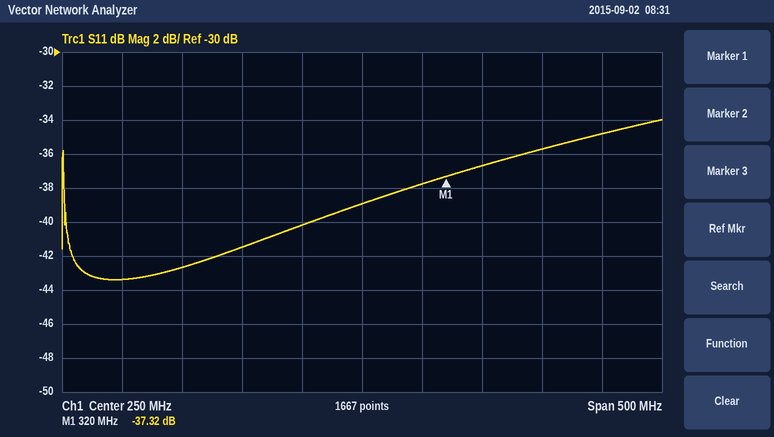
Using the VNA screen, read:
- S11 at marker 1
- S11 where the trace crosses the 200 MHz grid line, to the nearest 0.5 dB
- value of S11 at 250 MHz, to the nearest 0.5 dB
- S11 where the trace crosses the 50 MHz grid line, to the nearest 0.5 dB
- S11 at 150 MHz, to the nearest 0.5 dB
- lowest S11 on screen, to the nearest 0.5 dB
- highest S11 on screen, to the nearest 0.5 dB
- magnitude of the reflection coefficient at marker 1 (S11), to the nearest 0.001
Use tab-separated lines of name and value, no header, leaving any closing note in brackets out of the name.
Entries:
S11 at marker 1	-37.32 dB
S11 where the trace crosses the 200 MHz grid line, to the nearest 0.5 dB	-40.0 dB
value of S11 at 250 MHz, to the nearest 0.5 dB	-39.0 dB
S11 where the trace crosses the 50 MHz grid line, to the nearest 0.5 dB	-43.5 dB
S11 at 150 MHz, to the nearest 0.5 dB	-41.5 dB
lowest S11 on screen, to the nearest 0.5 dB	-43.5 dB
highest S11 on screen, to the nearest 0.5 dB	-34.0 dB
magnitude of the reflection coefficient at marker 1 (S11), to the nearest 0.001	0.014
